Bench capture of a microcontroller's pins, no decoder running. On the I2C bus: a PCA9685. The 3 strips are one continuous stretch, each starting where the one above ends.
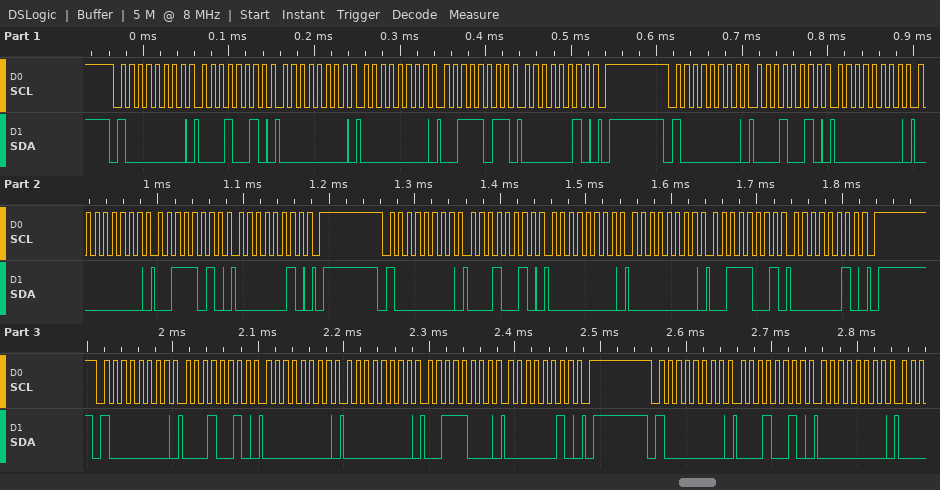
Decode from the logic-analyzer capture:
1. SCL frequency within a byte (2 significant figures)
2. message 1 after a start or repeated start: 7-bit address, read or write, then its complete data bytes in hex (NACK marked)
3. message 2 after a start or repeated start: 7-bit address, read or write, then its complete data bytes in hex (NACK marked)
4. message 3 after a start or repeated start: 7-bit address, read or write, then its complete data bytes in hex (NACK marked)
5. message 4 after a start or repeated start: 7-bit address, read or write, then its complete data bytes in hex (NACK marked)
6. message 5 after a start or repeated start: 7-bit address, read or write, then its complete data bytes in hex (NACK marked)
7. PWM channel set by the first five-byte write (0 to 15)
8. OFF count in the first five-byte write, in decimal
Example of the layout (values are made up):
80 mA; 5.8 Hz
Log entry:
100 kHz; 0x40 write: 12 00 00 3B 02; 0x40 write: 12 00 00 3A 02; 0x40 write: 12 00 00 39 02; 0x40 write: 12 00 00 38 02; 0x40 write: 12 00; 3; 571
